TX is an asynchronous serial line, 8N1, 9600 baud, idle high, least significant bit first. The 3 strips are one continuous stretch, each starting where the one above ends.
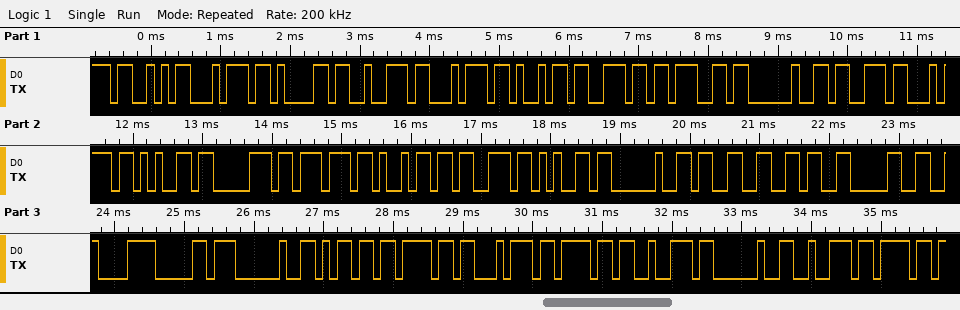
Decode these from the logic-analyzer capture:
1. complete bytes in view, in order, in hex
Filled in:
53 74 61 72 74 69 6E 67 20 73 74 65 70 77 69 73 65 20 33 36 30 C2 B0 20 6D 6F 74 6F 72 20 72 6F
